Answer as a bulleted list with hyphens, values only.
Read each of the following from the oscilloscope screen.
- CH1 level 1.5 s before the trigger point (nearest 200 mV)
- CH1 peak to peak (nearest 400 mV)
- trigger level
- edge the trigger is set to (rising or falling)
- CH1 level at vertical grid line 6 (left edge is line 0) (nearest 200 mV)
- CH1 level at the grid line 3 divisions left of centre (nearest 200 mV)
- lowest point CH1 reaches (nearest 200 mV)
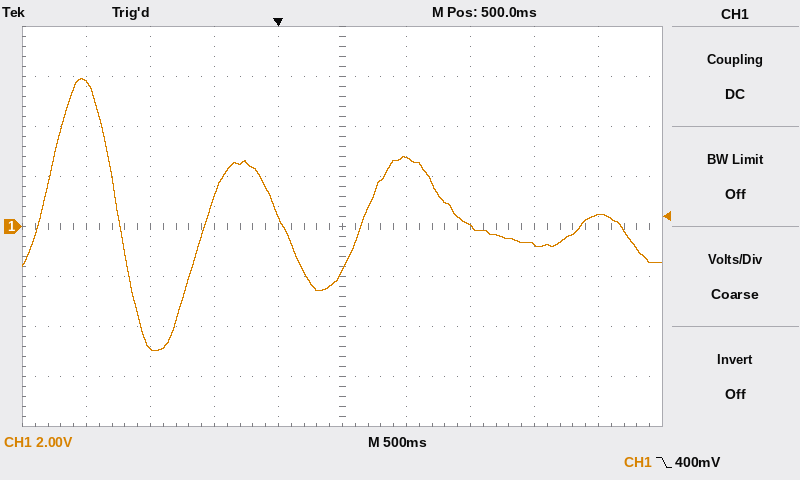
- 5.8 V
- 10.8 V
- 400 mV
- falling
- 2.8 V
- -4.8 V
- -5.0 V
